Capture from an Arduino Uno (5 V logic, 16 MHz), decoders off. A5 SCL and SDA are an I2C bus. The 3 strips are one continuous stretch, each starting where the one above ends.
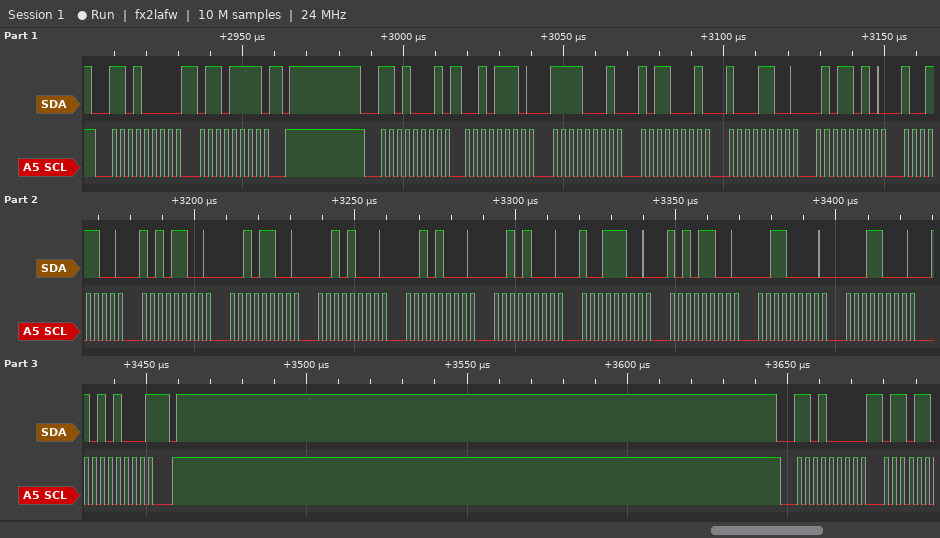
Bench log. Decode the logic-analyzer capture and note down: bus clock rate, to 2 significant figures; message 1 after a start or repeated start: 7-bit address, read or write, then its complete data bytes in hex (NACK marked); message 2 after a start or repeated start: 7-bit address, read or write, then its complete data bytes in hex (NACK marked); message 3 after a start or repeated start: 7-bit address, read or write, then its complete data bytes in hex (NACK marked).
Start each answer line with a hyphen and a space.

- 400 kHz
- 0x68 write: 6F
- 0x68 read: 2E F1 B1 8C 5A 9C AC 2C 28 28 28 9C AC 30 18 A8 NACK
- 0x68 write
